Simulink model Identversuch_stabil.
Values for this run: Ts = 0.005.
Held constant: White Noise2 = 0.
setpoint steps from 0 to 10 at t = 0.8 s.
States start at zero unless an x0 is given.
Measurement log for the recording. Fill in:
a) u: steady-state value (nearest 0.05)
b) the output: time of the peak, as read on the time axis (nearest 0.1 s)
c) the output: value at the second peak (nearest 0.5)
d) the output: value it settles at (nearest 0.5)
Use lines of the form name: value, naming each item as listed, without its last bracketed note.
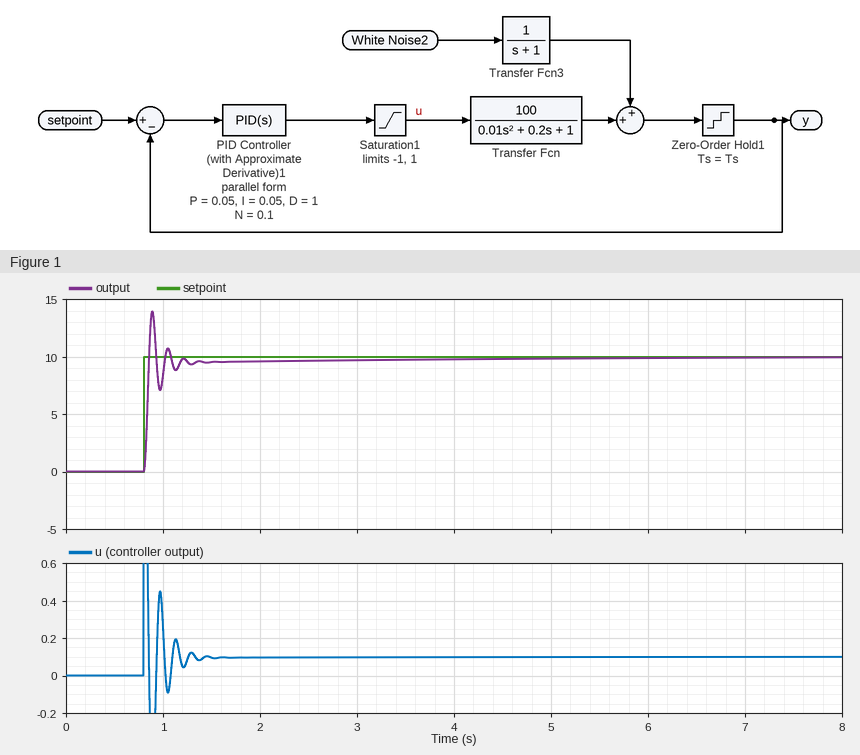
u: steady-state value: 0.10
the output: time of the peak, as read on the time axis: 0.9 s
the output: value at the second peak: 10.5
the output: value it settles at: 10.0
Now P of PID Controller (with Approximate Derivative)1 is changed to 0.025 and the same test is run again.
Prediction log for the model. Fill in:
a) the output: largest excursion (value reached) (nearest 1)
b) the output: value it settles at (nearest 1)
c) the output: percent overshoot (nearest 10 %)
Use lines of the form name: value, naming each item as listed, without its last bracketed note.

the output: largest excursion (value reached): 14
the output: value it settles at: 10
the output: percent overshoot: 40 %
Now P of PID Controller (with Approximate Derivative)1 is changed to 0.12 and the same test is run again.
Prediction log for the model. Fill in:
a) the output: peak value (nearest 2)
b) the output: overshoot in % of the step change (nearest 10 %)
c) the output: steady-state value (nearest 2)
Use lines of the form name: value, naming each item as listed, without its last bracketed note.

the output: peak value: 14
the output: overshoot in % of the step change: 40 %
the output: steady-state value: 10
